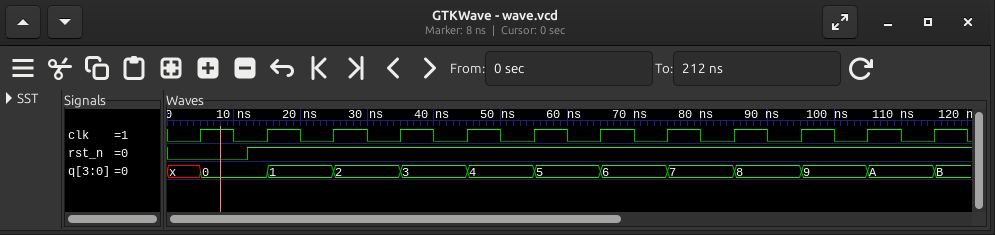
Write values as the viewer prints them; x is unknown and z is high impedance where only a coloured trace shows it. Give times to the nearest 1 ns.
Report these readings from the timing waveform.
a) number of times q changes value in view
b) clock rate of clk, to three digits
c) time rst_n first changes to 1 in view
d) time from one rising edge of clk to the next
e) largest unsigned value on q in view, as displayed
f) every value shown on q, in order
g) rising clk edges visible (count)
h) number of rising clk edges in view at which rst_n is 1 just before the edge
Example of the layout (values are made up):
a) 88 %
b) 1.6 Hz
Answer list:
a) 12
b) 100 MHz
c) 12 ns
d) 10 ns
e) B
f) x, 0, 1, 2, 3, 4, 5, 6, 7, 8, 9, A, B
g) 12
h) 11
